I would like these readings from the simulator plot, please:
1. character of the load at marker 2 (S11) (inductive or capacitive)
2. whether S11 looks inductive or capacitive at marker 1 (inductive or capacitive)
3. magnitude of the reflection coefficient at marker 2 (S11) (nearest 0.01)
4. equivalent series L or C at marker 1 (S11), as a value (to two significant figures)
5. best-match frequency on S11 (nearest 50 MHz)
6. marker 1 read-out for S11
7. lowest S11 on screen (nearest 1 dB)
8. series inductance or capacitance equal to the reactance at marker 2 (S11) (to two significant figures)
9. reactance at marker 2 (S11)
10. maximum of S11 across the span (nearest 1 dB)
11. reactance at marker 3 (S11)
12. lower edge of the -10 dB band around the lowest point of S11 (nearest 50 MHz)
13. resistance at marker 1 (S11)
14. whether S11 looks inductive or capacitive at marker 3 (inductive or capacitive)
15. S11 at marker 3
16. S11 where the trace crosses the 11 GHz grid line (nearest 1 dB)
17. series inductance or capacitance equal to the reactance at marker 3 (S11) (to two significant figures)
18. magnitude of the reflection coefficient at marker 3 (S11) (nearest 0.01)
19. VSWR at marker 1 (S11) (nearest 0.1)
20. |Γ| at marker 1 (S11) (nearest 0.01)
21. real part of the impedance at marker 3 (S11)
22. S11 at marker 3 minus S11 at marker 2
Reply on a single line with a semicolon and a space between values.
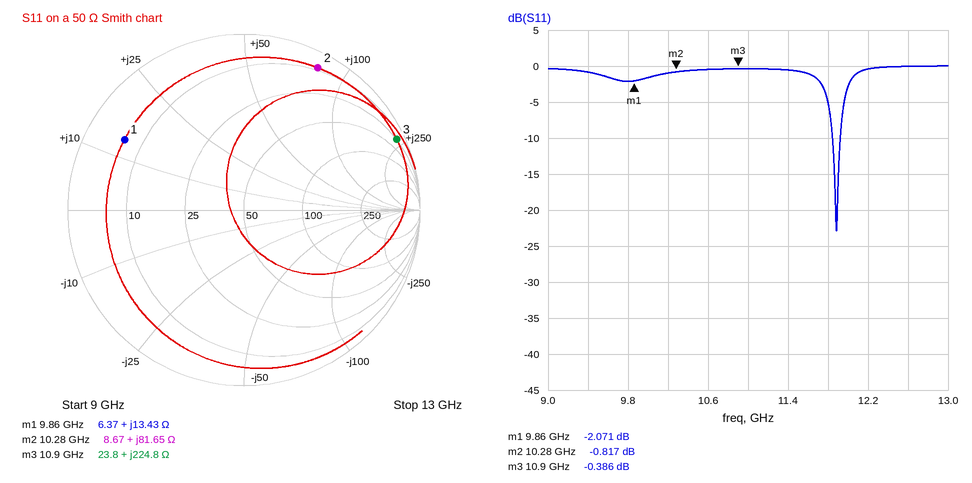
inductive; inductive; 0.91; 220 pH; 11.90 GHz; -2.071 dB; -23 dB; 1.3 nH; +81.65 Ω; 0 dB; +224.8 Ω; 11.85 GHz; 6.37 Ω; inductive; -0.386 dB; 0 dB; 3.3 nH; 0.96; 8.4; 0.79; 23.8 Ω; 0.431 dB
